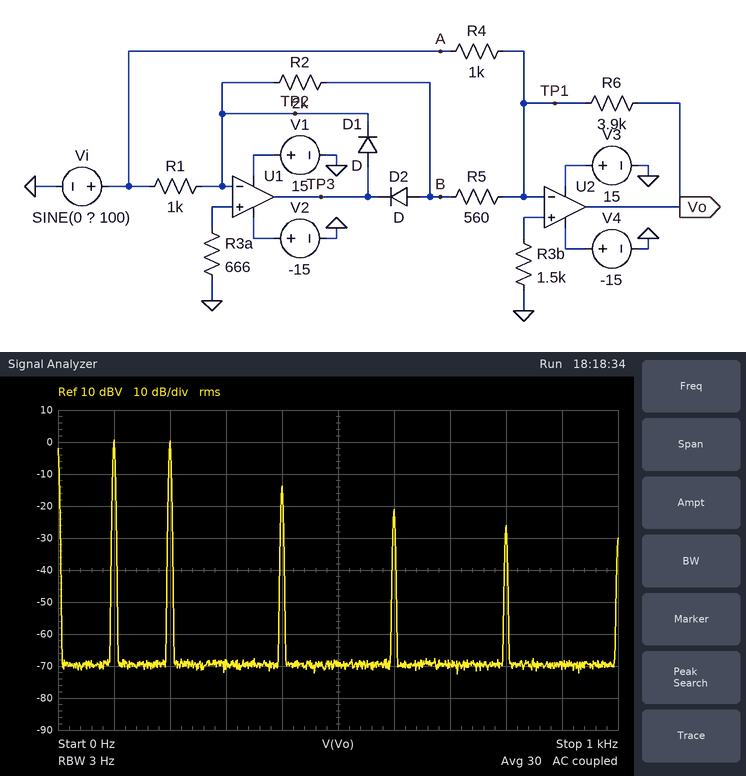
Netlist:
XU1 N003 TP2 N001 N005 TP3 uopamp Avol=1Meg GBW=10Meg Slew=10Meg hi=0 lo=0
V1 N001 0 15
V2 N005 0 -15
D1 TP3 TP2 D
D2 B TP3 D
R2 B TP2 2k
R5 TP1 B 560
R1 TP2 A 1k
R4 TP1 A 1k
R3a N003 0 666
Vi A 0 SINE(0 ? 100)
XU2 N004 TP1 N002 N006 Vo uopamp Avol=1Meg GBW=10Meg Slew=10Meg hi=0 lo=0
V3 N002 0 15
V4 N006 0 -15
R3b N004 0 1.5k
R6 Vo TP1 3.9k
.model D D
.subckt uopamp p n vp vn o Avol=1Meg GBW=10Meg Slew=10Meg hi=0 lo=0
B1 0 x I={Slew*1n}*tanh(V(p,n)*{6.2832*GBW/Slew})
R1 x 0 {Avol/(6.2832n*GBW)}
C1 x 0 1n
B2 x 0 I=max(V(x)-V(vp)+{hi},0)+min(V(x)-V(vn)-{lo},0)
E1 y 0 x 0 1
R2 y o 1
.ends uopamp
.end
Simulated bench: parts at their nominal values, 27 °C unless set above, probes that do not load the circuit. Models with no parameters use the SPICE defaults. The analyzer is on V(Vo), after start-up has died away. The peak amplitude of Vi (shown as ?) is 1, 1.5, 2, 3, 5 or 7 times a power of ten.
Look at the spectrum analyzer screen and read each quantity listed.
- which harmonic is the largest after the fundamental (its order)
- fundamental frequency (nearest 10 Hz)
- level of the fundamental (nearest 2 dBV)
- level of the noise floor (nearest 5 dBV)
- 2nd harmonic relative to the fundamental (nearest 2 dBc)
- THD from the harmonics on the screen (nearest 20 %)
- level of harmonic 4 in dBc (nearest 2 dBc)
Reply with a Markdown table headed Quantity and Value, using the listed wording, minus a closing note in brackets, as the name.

| Quantity | Value |
|---|---|
| which harmonic is the largest after the fundamental | 2 |
| fundamental frequency | 100 Hz |
| level of the fundamental | 0 dBV |
| level of the noise floor | -70 dBV |
| 2nd harmonic relative to the fundamental | 0 dBc |
| THD from the harmonics on the screen | 100 % |
| level of harmonic 4 in dBc | -14 dBc |
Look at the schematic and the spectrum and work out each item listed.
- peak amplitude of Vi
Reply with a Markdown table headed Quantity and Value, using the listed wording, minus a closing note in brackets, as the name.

| Quantity | Value |
|---|---|
| peak amplitude of Vi | 500 mV |
